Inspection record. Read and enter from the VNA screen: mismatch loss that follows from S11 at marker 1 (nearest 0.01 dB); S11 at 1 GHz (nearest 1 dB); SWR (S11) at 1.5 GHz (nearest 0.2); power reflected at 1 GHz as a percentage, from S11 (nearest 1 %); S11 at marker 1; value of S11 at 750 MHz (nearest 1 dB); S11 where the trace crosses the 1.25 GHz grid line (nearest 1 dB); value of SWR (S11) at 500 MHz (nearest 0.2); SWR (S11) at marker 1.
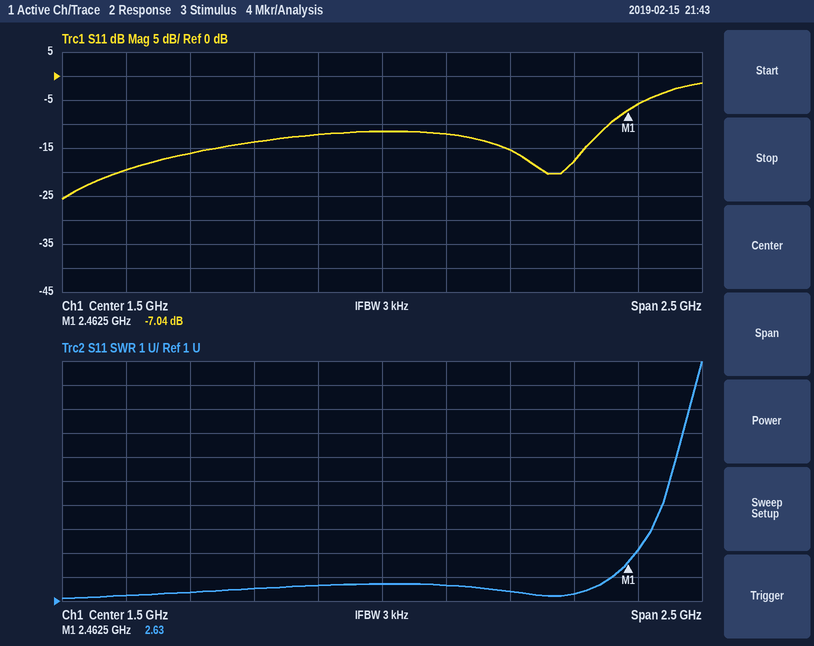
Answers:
0.96 dB
-14 dB
1.8
4 %
-7.04 dB
-16 dB
-12 dB
1.2
2.63
